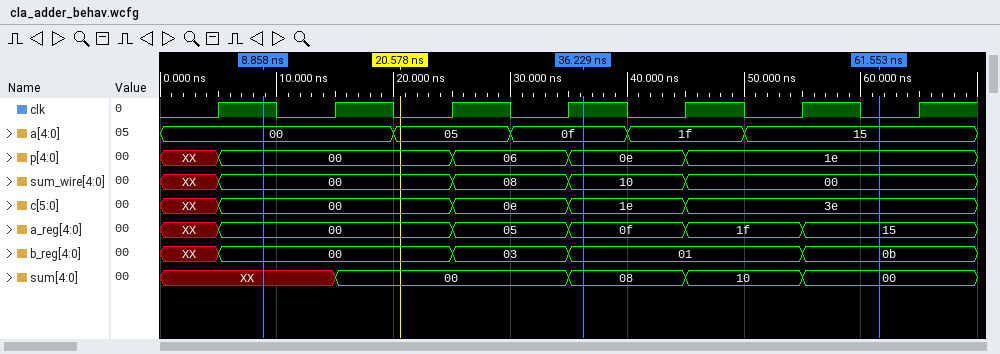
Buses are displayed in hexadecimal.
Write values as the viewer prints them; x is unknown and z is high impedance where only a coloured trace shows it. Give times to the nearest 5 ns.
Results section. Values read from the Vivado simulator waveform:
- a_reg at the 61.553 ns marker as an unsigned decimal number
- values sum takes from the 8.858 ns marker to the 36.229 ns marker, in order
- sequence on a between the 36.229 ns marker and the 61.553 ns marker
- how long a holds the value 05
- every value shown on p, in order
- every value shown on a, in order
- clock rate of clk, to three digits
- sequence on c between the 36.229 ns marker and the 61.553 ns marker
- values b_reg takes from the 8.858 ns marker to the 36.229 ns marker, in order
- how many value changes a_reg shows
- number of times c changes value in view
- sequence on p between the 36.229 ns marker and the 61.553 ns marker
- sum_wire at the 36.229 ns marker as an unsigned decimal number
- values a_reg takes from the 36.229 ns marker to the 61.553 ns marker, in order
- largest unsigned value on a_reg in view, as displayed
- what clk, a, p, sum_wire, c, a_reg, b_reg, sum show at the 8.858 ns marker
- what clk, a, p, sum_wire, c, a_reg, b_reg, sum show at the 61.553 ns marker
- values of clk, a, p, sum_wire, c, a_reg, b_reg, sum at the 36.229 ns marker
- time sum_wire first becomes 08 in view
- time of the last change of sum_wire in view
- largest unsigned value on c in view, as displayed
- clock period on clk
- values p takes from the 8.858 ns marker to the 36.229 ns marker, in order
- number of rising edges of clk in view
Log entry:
21
XX, 00, 08
0f, 1f, 15
10 ns
XX, 00, 06, 0e, 1e
00, 05, 0f, 1f, 15
100 MHz
1e, 3e
00, 03, 01
5
4
0e, 1e
16
0f, 1f, 15
1f
clk=1, a=00, p=00, sum_wire=00, c=00, a_reg=00, b_reg=00, sum=XX
clk=0, a=15, p=1e, sum_wire=00, c=3e, a_reg=15, b_reg=0b, sum=00
clk=1, a=0f, p=0e, sum_wire=10, c=1e, a_reg=0f, b_reg=01, sum=08
25 ns
45 ns
3e
10 ns
00, 06, 0e
7
